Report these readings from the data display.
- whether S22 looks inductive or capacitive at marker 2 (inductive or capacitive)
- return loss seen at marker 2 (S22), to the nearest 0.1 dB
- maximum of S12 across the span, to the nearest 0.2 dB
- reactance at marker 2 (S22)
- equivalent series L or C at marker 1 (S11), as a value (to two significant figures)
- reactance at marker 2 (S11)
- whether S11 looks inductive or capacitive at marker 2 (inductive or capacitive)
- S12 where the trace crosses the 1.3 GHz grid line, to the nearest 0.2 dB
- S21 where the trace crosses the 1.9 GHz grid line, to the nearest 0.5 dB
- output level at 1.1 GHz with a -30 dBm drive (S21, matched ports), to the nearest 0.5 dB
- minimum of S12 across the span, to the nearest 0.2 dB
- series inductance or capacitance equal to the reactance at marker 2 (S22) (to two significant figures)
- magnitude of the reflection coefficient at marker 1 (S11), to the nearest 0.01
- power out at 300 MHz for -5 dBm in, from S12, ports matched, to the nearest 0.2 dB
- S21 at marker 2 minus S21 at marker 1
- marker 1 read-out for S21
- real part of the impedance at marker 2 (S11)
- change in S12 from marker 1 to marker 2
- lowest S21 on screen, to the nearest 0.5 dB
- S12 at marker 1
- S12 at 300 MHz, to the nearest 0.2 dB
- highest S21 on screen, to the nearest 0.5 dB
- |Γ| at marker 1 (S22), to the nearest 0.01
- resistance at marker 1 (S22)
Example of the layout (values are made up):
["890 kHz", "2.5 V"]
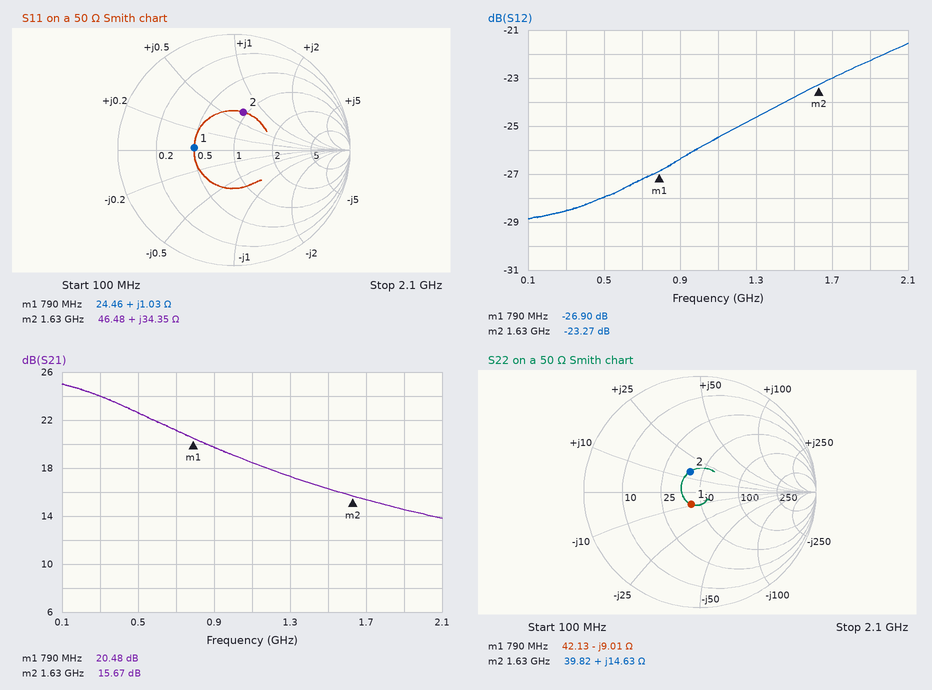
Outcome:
["inductive", "14.2 dB", "-21.6 dB", "+14.63 Ω", "210 pH", "+34.35 Ω", "inductive", "-24.6 dB", "14.5 dB", "-11.5 dBm", "-28.8 dB", "1.4 nH", "0.34", "-33.6 dBm", "-4.81 dB", "20.48 dB", "46.48 Ω", "3.63 dB", "14.0 dB", "-26.90 dB", "-28.6 dB", "25.0 dB", "0.13", "42.13 Ω"]
